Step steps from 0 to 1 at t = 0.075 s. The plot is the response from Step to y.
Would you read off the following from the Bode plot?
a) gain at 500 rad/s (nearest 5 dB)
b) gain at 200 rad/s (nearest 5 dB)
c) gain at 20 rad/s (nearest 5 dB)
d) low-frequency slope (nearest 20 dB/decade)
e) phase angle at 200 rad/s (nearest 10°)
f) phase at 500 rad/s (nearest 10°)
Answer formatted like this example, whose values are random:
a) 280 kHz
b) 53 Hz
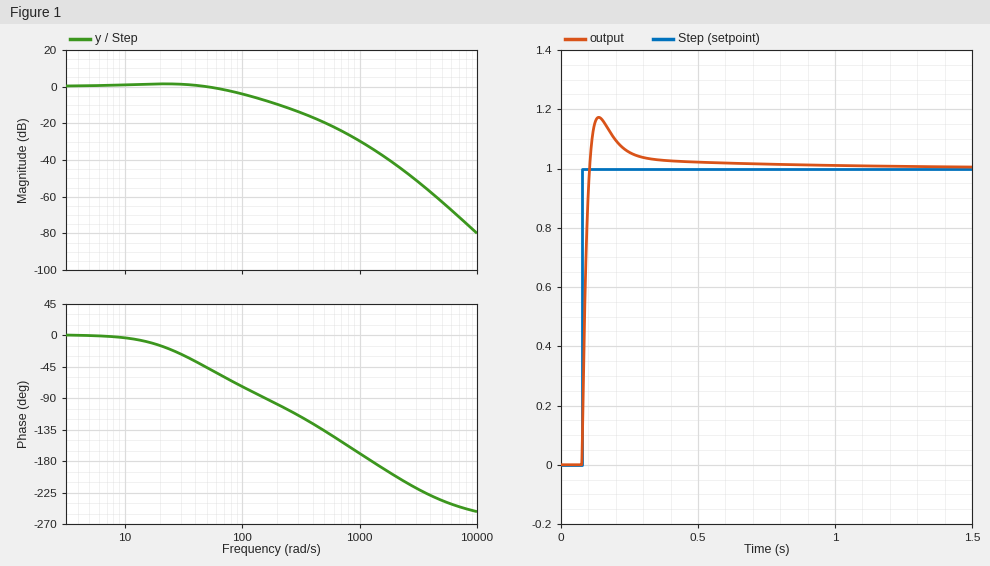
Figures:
a) -20 dB
b) -10 dB
c) 0 dB
d) 0 dB/decade
e) -100°
f) -140°
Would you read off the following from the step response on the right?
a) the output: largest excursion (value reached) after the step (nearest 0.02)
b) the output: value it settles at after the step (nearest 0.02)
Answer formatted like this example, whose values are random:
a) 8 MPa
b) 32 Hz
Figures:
a) 1.18
b) 1.00
